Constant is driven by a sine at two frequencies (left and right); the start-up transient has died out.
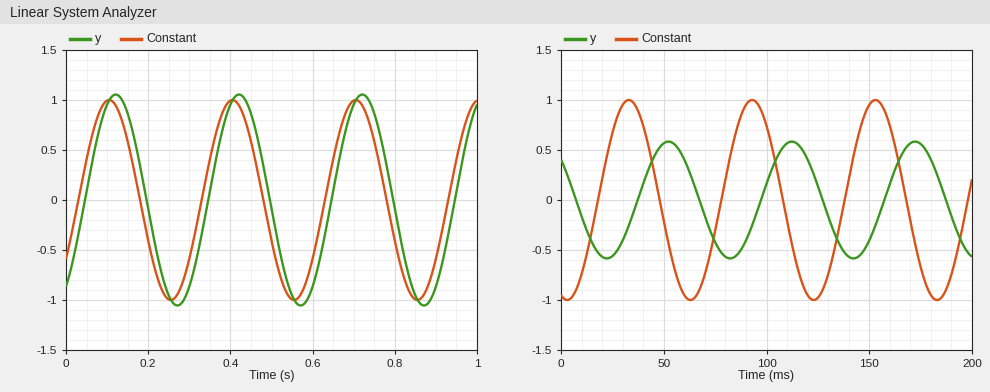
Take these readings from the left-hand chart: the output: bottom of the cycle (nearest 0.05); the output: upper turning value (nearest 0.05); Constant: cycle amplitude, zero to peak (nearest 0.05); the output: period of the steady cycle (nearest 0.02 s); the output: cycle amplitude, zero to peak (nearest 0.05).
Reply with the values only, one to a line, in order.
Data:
-1.05
1.05
1.00
0.30 s
1.05
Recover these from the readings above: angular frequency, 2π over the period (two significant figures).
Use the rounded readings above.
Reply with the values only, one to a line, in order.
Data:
21 rad/s
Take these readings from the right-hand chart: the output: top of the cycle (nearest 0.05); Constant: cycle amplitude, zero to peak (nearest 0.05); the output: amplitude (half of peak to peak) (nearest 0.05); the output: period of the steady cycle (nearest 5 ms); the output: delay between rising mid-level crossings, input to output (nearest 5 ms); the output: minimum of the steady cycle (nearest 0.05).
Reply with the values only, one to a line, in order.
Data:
0.60
1.00
0.60
60 ms
20 ms
-0.60
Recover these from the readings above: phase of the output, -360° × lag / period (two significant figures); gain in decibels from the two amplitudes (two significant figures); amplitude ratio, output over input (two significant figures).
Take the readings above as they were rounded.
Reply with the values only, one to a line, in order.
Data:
-120°
-4.4 dB
0.60
